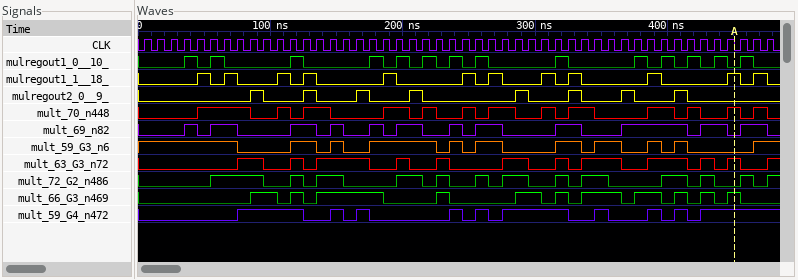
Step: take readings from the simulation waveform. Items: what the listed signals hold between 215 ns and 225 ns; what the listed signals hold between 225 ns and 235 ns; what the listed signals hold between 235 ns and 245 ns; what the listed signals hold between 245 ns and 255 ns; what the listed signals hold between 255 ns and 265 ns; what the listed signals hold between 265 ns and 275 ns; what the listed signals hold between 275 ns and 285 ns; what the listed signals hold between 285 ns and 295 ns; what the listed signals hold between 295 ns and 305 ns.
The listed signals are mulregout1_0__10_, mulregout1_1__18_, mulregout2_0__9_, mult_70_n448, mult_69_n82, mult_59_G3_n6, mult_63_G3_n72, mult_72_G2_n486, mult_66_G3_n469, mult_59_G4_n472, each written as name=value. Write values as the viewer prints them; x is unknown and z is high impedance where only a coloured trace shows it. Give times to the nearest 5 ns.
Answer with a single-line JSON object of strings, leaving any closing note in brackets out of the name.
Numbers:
{"what the listed signals hold between 215 ns and 225 ns": "mulregout1_0__10_=1, mulregout1_1__18_=0, mulregout2_0__9_=0, mult_70_n448=1, mult_69_n82=0, mult_59_G3_n6=1, mult_63_G3_n72=0, mult_72_G2_n486=0, mult_66_G3_n469=0, mult_59_G4_n472=0", "what the listed signals hold between 225 ns and 235 ns": "mulregout1_0__10_=0, mulregout1_1__18_=0, mulregout2_0__9_=0, mult_70_n448=0, mult_69_n82=0, mult_59_G3_n6=0, mult_63_G3_n72=1, mult_72_G2_n486=1, mult_66_G3_n469=1, mult_59_G4_n472=0", "what the listed signals hold between 235 ns and 245 ns": "mulregout1_0__10_=1, mulregout1_1__18_=0, mulregout2_0__9_=0, mult_70_n448=0, mult_69_n82=1, mult_59_G3_n6=1, mult_63_G3_n72=0, mult_72_G2_n486=0, mult_66_G3_n469=0, mult_59_G4_n472=1", "what the listed signals hold between 245 ns and 255 ns": "mulregout1_0__10_=0, mulregout1_1__18_=1, mulregout2_0__9_=0, mult_70_n448=1, mult_69_n82=0, mult_59_G3_n6=0, mult_63_G3_n72=0, mult_72_G2_n486=0, mult_66_G3_n469=0, mult_59_G4_n472=0", "what the listed signals hold between 255 ns and 265 ns": "mulregout1_0__10_=1, mulregout1_1__18_=0, mulregout2_0__9_=0, mult_70_n448=0, mult_69_n82=1, mult_59_G3_n6=1, mult_63_G3_n72=0, mult_72_G2_n486=1, mult_66_G3_n469=0, mult_59_G4_n472=1", "what the listed signals hold between 265 ns and 275 ns": "mulregout1_0__10_=0, mulregout1_1__18_=1, mulregout2_0__9_=0, mult_70_n448=1, mult_69_n82=1, mult_59_G3_n6=1, mult_63_G3_n72=0, mult_72_G2_n486=0, mult_66_G3_n469=0, mult_59_G4_n472=0", "what the listed signals hold between 275 ns and 285 ns": "mulregout1_0__10_=0, mulregout1_1__18_=0, mulregout2_0__9_=0, mult_70_n448=1, mult_69_n82=0, mult_59_G3_n6=0, mult_63_G3_n72=1, mult_72_G2_n486=1, mult_66_G3_n469=0, mult_59_G4_n472=1", "what the listed signals hold between 285 ns and 295 ns": "mulregout1_0__10_=0, mulregout1_1__18_=0, mulregout2_0__9_=1, mult_70_n448=0, mult_69_n82=0, mult_59_G3_n6=0, mult_63_G3_n72=1, mult_72_G2_n486=1, mult_66_G3_n469=1, mult_59_G4_n472=1", "what the listed signals hold between 295 ns and 305 ns": "mulregout1_0__10_=0, mulregout1_1__18_=0, mulregout2_0__9_=0, mult_70_n448=0, mult_69_n82=0, mult_59_G3_n6=0, mult_63_G3_n72=0, mult_72_G2_n486=0, mult_66_G3_n469=1, mult_59_G4_n472=1"}
